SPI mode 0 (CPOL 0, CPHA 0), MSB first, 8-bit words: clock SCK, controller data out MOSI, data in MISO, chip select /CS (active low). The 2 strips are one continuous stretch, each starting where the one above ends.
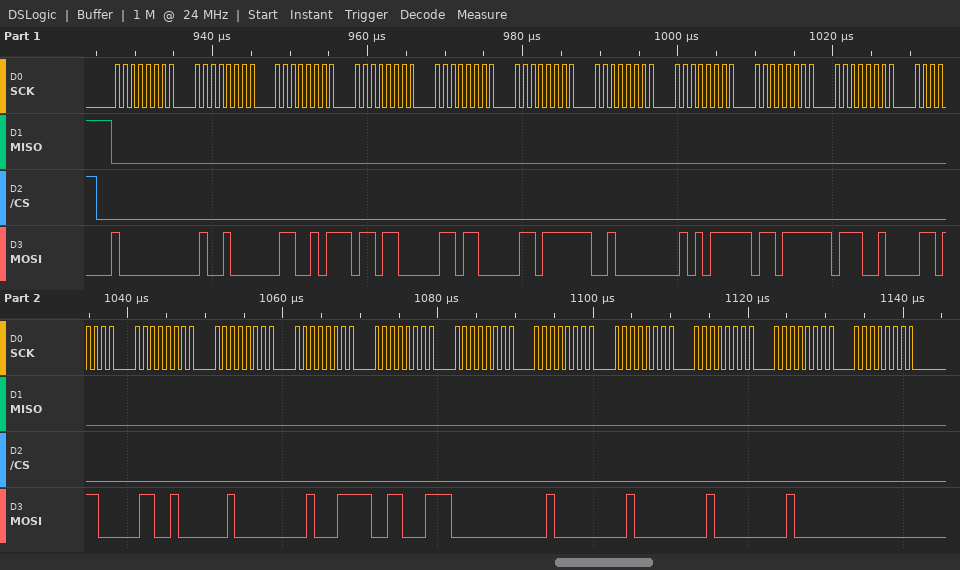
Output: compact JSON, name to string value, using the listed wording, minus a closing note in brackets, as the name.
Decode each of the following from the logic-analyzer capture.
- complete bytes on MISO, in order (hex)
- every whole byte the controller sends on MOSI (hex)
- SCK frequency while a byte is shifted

{"complete bytes on MISO, in order": "0x00 0x00 0x00 0x00 0x00 0x00 0x00 0x00 0x00 0x00 0x00 0x00 0x00 0x00 0x00 0x00 0x00 0x00 0x00 0x00 0x00", "every whole byte the controller sends on MOSI": "0x80 0x48 0x65 0x6C 0x6C 0x6F 0x20 0x57 0x6F 0x72 0x6C 0x64 0x20 0x23 0x31 0x00 0x20 0x20 0x20 0x20 0x00", "SCK frequency while a byte is shifted": "1 MHz"}
